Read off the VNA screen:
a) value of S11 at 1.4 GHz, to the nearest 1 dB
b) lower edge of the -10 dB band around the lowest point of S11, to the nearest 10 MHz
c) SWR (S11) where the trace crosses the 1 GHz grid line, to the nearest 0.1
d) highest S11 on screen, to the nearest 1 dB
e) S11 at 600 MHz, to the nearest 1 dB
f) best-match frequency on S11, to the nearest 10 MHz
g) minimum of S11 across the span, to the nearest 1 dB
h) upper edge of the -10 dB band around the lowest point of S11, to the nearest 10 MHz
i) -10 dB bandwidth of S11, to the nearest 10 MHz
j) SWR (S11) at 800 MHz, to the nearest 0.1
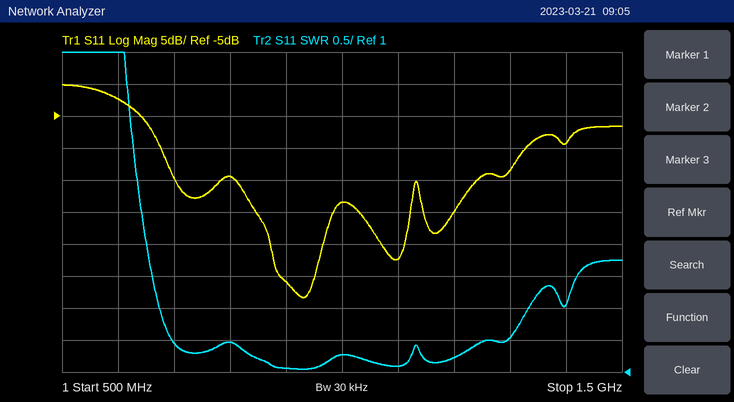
-9 dB
680 MHz
1.3
0 dB
-2 dB
930 MHz
-33 dB
1.33 GHz
650 MHz
1.5
